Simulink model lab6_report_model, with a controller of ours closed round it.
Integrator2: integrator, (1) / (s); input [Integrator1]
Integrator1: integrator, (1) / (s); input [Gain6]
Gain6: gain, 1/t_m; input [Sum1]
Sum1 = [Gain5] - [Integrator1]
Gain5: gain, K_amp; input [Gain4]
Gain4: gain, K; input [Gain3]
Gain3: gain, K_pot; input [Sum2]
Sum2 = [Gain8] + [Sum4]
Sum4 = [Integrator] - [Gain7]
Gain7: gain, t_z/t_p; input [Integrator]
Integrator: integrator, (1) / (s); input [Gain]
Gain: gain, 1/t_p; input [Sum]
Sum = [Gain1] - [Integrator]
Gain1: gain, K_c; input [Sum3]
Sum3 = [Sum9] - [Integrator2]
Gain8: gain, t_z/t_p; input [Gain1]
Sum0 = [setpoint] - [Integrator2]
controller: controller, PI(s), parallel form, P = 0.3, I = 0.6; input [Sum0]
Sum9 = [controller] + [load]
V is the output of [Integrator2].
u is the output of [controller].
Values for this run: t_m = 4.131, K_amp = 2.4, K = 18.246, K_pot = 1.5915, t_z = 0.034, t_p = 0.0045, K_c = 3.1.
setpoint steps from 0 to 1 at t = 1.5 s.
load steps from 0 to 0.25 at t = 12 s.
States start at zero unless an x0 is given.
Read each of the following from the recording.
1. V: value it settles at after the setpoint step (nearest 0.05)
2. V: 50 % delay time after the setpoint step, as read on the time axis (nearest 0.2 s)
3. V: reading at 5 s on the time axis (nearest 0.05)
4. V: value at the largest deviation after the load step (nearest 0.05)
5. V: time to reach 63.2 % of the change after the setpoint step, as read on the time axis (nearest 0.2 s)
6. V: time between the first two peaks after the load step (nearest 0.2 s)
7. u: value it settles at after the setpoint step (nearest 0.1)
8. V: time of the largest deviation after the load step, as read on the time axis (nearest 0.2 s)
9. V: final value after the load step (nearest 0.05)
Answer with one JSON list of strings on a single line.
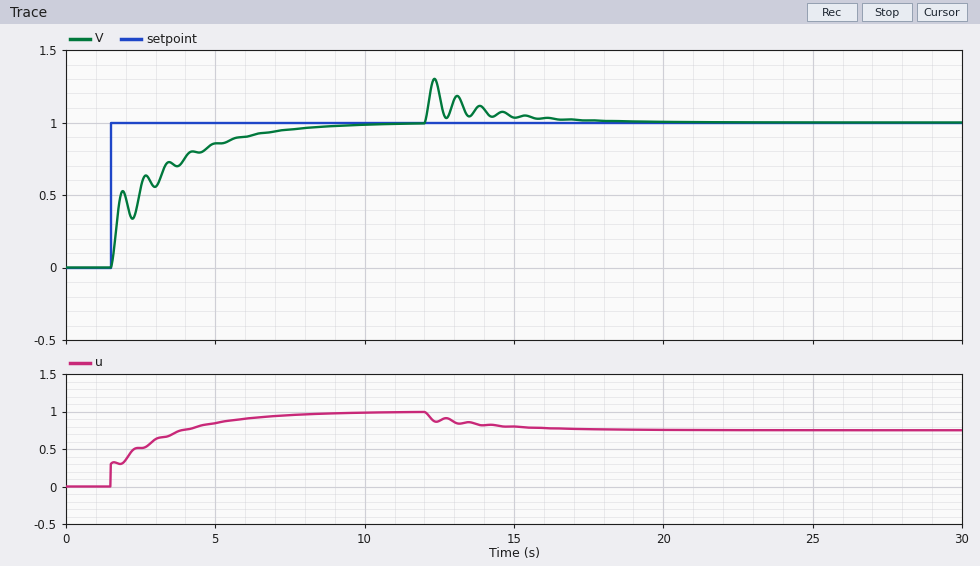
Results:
["1.00", "1.8 s", "0.85", "1.30", "2.6 s", "0.8 s", "1.0", "12.4 s", "1.00"]
